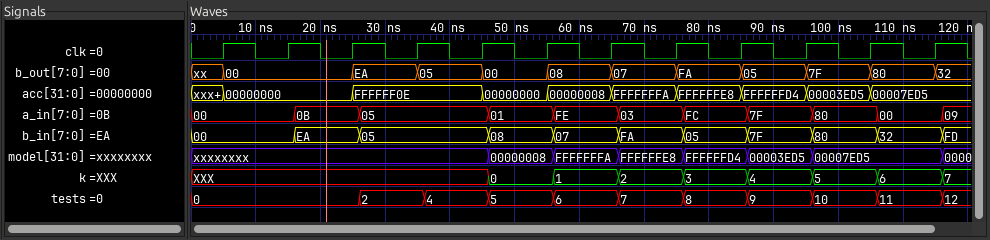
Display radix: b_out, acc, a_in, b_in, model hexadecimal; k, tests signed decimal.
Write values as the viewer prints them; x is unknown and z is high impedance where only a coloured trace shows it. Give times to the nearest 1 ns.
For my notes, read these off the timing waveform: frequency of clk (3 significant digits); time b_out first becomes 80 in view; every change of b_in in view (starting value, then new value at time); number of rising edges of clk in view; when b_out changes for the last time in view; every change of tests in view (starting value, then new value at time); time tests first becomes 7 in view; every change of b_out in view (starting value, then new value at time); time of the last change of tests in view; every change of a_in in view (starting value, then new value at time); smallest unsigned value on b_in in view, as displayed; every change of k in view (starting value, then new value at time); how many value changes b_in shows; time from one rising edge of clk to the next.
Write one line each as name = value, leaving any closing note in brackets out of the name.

frequency of clk = 100 MHz
time b_out first becomes 80 in view = 105 ns
every change of b_in in view = 00, EA at 16 ns, 05 at 26 ns, 08 at 46 ns, 07 at 56 ns, FA at 66 ns, 05 at 76 ns, 7F at 86 ns, 80 at 96 ns, 32 at 106 ns, FD at 116 ns
number of rising edges of clk in view = 12
when b_out changes for the last time in view = 115 ns
every change of tests in view = 0, 2 at 26 ns, 4 at 36 ns, 5 at 46 ns, 6 at 56 ns, 7 at 66 ns, 8 at 76 ns, 9 at 86 ns, 10 at 96 ns, 11 at 106 ns, 12 at 116 ns
time tests first becomes 7 in view = 66 ns
every change of b_out in view = xx, 00 at 5 ns, EA at 25 ns, 05 at 35 ns, 00 at 45 ns, 08 at 55 ns, 07 at 65 ns, FA at 75 ns, 05 at 85 ns, 7F at 95 ns, 80 at 105 ns, 32 at 115 ns
time of the last change of tests in view = 116 ns
every change of a_in in view = 00, 0B at 16 ns, 05 at 26 ns, 01 at 46 ns, FE at 56 ns, 03 at 66 ns, FC at 76 ns, 7F at 86 ns, 80 at 96 ns, 00 at 106 ns, 09 at 116 ns
smallest unsigned value on b_in in view, as displayed = 00
every change of k in view = XXX, 0 at 46 ns, 1 at 56 ns, 2 at 66 ns, 3 at 76 ns, 4 at 86 ns, 5 at 96 ns, 6 at 106 ns, 7 at 116 ns
how many value changes b_in shows = 10
time from one rising edge of clk to the next = 10 ns
